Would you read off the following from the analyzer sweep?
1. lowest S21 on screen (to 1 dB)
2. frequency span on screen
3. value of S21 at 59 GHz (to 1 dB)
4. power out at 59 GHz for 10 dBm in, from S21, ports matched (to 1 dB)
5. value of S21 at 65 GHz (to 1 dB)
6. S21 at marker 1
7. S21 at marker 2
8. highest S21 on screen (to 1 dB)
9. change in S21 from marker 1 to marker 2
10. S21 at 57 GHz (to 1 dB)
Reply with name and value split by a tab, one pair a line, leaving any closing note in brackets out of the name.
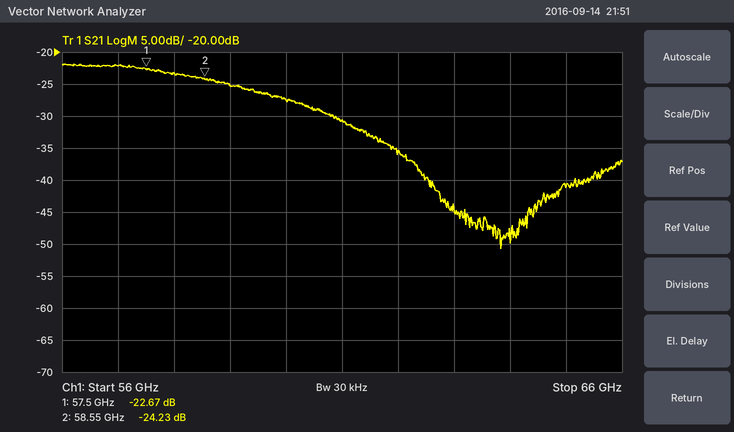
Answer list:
lowest S21 on screen	-51 dB
frequency span on screen	10 GHz
value of S21 at 59 GHz	-25 dB
power out at 59 GHz for 10 dBm in, from S21, ports matched	-15 dBm
value of S21 at 65 GHz	-41 dB
S21 at marker 1	-22.67 dB
S21 at marker 2	-24.23 dB
highest S21 on screen	-22 dB
change in S21 from marker 1 to marker 2	-1.56 dB
S21 at 57 GHz	-22 dB
